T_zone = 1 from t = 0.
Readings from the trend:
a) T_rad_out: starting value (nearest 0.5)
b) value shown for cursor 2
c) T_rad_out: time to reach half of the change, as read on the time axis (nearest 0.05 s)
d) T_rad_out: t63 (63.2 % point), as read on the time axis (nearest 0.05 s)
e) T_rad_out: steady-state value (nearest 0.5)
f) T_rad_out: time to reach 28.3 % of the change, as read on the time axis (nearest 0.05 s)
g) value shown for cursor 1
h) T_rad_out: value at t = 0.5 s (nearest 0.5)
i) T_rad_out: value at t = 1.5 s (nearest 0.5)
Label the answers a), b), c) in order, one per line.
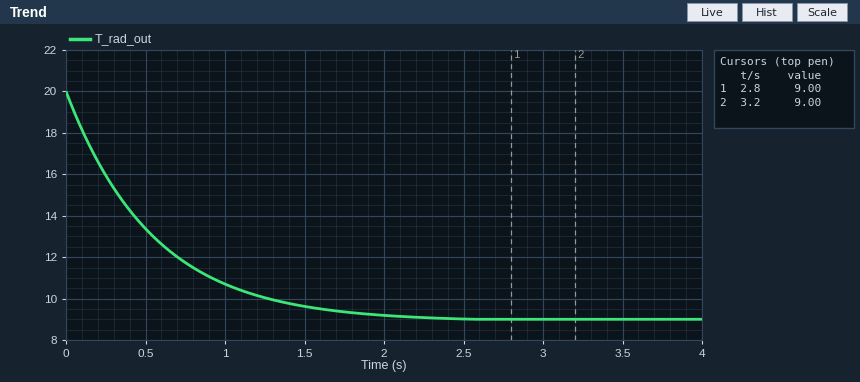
a) 20.0
b) 9.00
c) 0.40 s
d) 0.55 s
e) 9.0
f) 0.20 s
g) 9.00
h) 13.5
i) 9.5
